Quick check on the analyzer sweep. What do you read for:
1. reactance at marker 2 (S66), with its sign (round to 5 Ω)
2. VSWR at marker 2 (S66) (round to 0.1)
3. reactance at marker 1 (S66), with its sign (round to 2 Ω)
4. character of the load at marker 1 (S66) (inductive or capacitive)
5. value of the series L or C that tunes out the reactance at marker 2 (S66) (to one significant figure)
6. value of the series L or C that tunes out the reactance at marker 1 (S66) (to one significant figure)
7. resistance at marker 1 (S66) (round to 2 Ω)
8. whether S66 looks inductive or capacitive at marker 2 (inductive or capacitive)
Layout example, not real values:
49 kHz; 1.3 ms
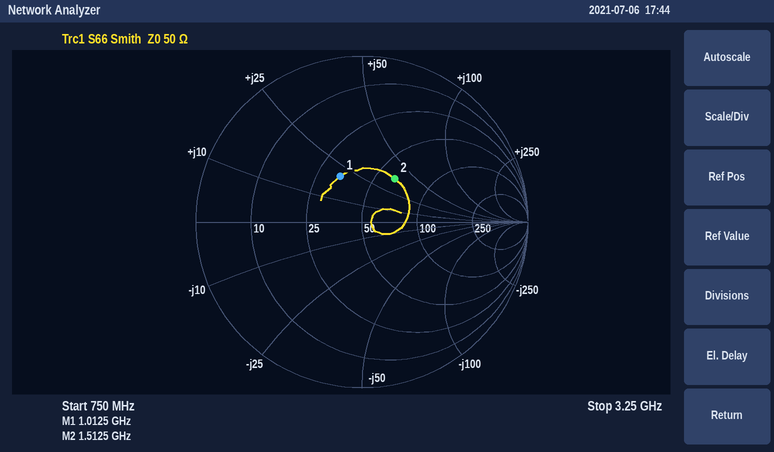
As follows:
+35 Ω; 2.0; +20 Ω; inductive; 3 pF; 8 pF; 34 Ω; inductive
